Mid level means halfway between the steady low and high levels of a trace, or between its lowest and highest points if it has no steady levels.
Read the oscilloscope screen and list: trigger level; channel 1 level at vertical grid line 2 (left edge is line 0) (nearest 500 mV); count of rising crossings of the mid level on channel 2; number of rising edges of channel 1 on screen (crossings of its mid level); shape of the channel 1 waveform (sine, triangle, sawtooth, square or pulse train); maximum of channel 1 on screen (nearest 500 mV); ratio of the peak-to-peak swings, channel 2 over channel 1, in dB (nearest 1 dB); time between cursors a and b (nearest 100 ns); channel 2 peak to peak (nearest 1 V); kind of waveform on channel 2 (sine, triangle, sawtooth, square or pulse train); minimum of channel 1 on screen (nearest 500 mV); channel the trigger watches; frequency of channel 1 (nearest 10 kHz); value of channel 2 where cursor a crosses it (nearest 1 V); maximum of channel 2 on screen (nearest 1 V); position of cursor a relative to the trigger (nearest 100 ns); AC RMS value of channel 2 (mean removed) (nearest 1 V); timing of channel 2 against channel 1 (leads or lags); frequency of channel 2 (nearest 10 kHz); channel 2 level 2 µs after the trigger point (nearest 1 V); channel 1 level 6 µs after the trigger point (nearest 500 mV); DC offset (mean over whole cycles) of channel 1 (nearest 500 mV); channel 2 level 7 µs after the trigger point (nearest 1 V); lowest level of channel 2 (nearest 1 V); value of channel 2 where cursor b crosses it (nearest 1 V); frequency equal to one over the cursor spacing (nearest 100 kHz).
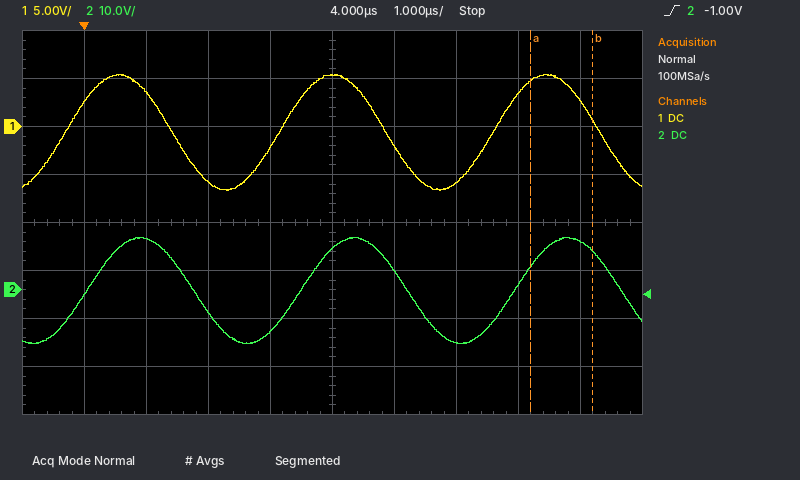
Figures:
-1.00 V
3.5 V
3
3
sine
5.5 V
5 dB
1.0 µs
22 V
sine
-6.5 V
channel 2
290 kHz
5 V
11 V
+7.2 µs
8 V
lags
290 kHz
-5 V
-6.0 V
-500 mV
1 V
-11 V
8 V
1.0 MHz
